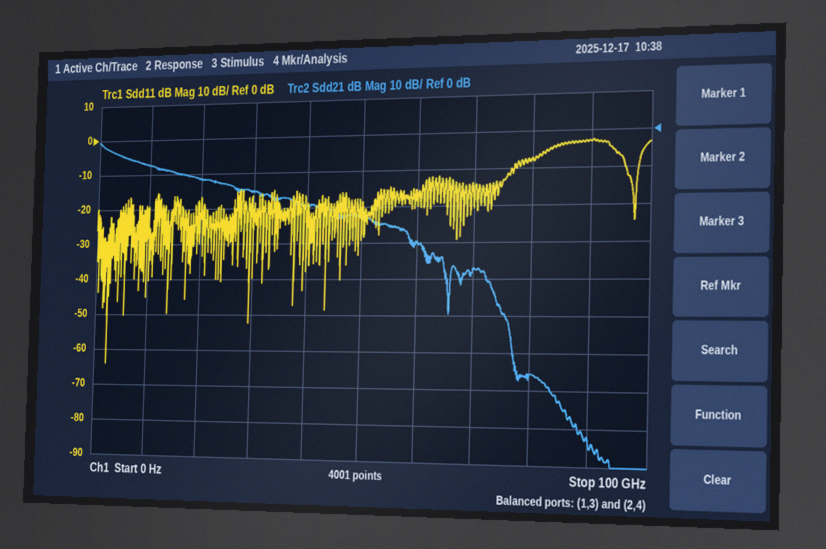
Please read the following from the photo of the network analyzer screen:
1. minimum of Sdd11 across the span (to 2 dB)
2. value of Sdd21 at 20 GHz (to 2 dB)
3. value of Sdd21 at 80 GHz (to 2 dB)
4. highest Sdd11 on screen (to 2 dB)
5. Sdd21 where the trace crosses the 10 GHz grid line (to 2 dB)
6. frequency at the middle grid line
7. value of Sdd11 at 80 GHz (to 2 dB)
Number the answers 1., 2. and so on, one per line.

1. -64 dB
2. -12 dB
3. -66 dB
4. -2 dB
5. -8 dB
6. 50 GHz
7. -8 dB
